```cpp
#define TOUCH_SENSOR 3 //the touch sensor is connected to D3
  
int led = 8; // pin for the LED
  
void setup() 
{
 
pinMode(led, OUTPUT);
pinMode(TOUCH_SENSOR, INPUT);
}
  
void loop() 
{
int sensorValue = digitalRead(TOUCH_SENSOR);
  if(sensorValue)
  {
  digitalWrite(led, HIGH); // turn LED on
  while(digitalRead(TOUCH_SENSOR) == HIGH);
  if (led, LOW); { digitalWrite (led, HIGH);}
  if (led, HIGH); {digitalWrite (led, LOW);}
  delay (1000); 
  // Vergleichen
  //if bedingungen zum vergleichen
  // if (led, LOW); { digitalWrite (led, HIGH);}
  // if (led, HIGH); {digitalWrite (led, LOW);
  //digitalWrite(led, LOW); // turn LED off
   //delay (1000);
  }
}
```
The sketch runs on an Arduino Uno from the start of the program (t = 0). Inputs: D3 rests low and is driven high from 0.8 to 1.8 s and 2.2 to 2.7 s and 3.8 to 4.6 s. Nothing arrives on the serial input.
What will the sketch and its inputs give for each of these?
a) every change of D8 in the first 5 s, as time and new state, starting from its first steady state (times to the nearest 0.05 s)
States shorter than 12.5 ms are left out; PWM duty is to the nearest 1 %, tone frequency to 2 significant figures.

0 s low; 0.8 s high; 1.8 s low; 3.8 s high; 4.6 s low
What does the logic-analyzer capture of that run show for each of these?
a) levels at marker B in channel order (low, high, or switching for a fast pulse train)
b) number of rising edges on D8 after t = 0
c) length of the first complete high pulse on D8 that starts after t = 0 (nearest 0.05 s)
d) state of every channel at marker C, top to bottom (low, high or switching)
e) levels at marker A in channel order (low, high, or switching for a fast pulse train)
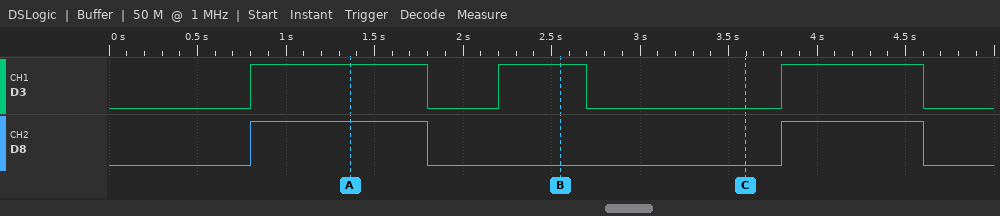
D3 high, D8 low
2
1.00 s
D3 low, D8 low
D3 high, D8 high
